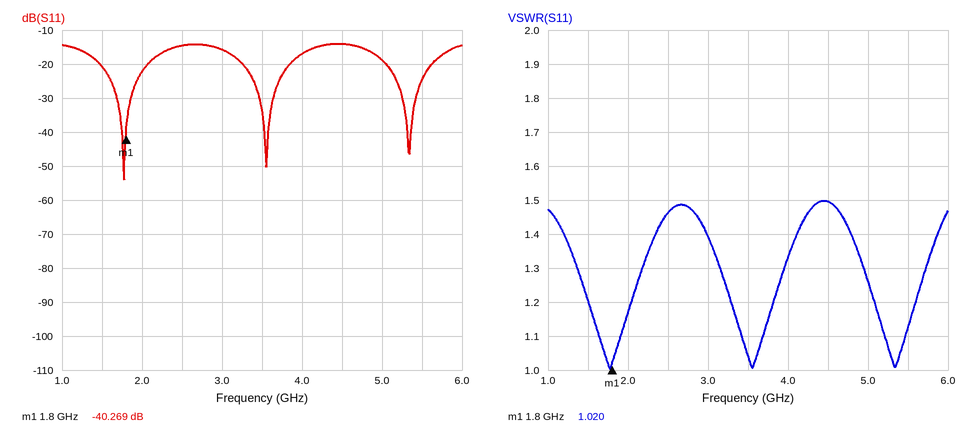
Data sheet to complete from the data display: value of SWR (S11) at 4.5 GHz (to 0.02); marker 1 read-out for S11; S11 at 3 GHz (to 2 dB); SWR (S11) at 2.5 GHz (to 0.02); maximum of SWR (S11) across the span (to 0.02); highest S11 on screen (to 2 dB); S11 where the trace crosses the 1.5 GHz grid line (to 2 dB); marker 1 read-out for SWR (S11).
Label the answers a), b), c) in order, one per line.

a) 1.50
b) -40.269 dB
c) -16 dB
d) 1.46
e) 1.50
f) -14 dB
g) -20 dB
h) 1.020
